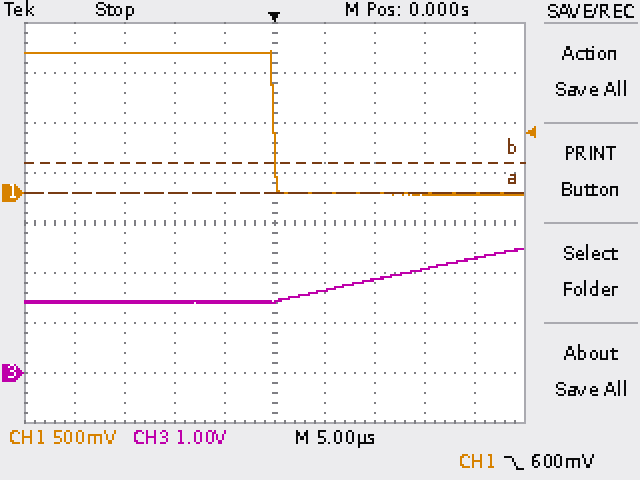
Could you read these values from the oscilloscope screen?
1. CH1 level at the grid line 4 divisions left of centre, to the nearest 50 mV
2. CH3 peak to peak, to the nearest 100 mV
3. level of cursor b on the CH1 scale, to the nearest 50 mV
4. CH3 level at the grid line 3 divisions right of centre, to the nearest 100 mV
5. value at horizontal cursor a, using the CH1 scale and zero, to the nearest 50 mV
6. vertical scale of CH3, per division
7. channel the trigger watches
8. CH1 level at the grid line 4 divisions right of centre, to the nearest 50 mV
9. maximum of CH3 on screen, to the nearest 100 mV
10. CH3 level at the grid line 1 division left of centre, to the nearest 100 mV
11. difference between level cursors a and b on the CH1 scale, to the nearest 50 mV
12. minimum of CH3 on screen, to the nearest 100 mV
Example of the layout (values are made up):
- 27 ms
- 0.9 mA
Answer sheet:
- 1.40 V
- 1.1 V
- 300 mV
- 2.1 V
- 0 mV
- 1 V
- CH1
- 0 mV
- 2.5 V
- 1.4 V
- 300 mV
- 1.4 V
